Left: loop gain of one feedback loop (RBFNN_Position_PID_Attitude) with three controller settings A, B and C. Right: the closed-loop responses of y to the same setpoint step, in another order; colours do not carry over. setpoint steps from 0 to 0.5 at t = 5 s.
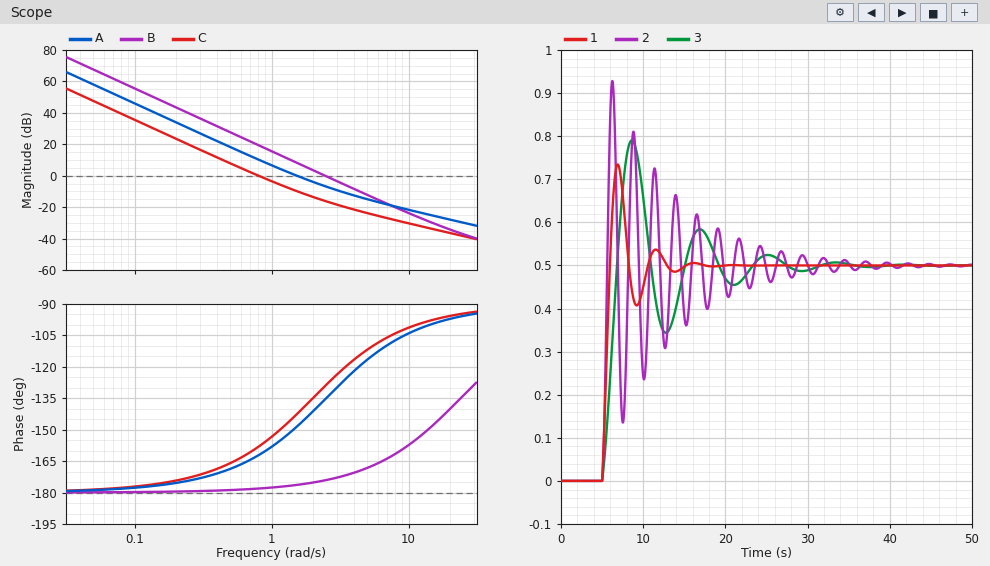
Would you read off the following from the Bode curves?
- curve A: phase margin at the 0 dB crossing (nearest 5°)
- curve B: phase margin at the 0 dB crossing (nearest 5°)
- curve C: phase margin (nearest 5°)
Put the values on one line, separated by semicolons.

30°; 5°; 20°
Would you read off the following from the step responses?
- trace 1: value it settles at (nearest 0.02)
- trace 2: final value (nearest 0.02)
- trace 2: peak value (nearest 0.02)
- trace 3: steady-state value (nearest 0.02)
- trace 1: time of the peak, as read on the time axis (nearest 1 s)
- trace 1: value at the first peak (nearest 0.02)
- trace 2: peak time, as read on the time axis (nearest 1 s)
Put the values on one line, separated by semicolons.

0.50; 0.50; 0.92; 0.50; 7 s; 0.74; 6 s
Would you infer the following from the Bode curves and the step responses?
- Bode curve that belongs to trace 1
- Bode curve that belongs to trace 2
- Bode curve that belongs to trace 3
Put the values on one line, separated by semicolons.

A; B; C
